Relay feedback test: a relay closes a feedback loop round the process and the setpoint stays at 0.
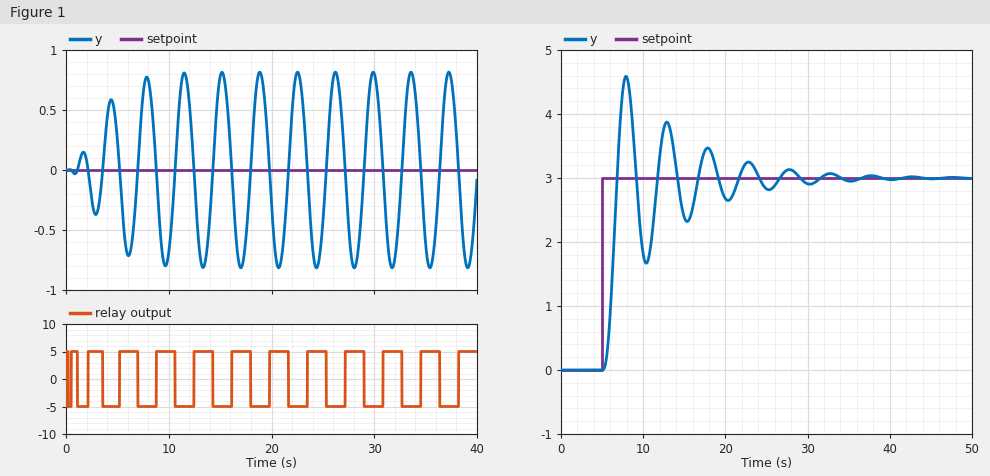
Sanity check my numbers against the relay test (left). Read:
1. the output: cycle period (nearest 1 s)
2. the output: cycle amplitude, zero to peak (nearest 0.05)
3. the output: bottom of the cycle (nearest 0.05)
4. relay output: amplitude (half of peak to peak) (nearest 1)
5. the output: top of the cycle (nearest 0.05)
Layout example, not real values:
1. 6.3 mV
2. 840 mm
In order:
1. 4 s
2. 0.80
3. -0.80
4. 5
5. 0.80
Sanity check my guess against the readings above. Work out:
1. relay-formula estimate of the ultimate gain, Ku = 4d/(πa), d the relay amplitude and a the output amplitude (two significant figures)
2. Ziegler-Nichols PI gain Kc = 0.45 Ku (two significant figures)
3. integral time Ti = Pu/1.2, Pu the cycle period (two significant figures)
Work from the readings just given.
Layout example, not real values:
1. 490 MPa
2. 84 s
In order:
1. 8.0
2. 3.6
3. 3.3 s
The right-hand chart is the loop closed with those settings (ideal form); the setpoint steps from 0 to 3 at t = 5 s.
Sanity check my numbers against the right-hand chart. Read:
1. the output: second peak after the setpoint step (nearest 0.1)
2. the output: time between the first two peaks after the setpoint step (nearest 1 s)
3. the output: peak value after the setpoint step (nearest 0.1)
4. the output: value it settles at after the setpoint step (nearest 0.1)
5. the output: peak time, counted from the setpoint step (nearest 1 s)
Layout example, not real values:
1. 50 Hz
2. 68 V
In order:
1. 3.9
2. 5 s
3. 4.6
4. 3.0
5. 3 s
